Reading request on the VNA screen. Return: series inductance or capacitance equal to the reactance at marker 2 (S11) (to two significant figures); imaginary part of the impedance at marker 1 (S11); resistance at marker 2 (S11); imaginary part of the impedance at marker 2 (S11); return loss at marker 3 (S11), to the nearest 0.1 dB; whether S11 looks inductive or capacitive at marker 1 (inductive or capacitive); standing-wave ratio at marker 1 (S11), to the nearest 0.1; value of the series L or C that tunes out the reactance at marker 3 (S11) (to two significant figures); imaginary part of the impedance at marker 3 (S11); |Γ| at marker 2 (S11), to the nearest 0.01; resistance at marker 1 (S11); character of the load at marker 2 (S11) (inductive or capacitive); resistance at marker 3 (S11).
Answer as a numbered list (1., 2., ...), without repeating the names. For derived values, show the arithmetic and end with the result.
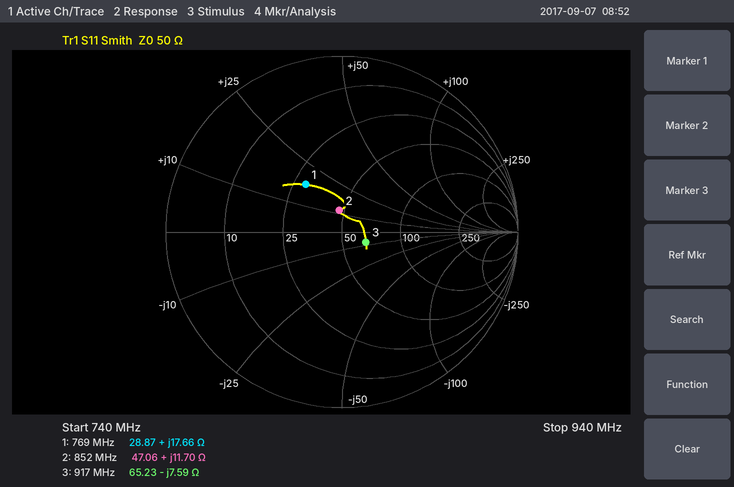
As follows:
1. L = 11.7 Ω/(2π × 852 MHz) ≈ 2.2 nH
2. +17.66 Ω
3. 47.06 Ω
4. +11.70 Ω
5. 16.6 dB
6. inductive
7. 2.0
8. L = 7.59 Ω/(2π × 917 MHz) ≈ 1.3 nH
9. -7.59 Ω
10. 0.12
11. 28.87 Ω
12. inductive
13. 65.23 Ω
